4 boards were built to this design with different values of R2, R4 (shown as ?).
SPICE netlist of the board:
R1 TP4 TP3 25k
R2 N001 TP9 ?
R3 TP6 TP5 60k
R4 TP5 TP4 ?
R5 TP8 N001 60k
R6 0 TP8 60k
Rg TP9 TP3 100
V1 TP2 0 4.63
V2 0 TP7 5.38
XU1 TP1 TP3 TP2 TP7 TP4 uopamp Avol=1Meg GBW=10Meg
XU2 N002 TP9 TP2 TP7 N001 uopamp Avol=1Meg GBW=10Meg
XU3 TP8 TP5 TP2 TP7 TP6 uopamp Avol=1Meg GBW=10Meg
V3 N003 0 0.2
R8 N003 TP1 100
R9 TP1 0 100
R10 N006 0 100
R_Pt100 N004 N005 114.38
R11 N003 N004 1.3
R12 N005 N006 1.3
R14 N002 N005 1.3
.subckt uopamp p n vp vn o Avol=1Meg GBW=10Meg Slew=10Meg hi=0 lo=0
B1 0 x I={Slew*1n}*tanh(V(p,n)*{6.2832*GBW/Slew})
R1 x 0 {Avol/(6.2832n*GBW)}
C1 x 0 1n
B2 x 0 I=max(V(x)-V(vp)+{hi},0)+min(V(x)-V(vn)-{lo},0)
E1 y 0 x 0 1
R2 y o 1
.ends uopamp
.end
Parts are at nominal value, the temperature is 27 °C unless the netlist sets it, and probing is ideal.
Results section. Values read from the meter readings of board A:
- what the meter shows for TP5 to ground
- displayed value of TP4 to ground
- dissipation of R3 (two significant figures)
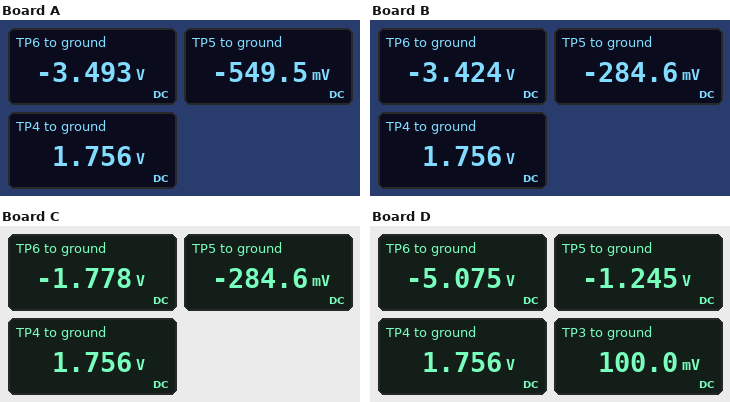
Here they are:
-549.5 mV
1.756 V
140 µW
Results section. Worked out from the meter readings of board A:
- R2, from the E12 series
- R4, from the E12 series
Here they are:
18 kΩ
47 kΩ
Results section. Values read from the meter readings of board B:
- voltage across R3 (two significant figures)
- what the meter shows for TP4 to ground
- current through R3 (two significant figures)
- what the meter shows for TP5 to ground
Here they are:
3.1 V
1.756 V
52 µA
-284.6 mV
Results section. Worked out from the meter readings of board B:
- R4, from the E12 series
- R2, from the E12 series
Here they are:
39 kΩ
10 kΩ
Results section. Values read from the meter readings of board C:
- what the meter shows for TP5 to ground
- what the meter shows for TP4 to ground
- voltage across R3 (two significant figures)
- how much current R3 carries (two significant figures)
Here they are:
-284.6 mV
1.756 V
1.5 V
25 µA
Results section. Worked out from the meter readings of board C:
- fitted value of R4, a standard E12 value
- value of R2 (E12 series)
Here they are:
82 kΩ
10 kΩ
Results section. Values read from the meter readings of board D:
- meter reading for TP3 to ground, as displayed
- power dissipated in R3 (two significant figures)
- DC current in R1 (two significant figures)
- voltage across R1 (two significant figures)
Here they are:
100.0 mV
240 µW
66 µA
1.7 V
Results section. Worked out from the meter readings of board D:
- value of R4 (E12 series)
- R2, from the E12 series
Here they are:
47 kΩ
39 kΩ
